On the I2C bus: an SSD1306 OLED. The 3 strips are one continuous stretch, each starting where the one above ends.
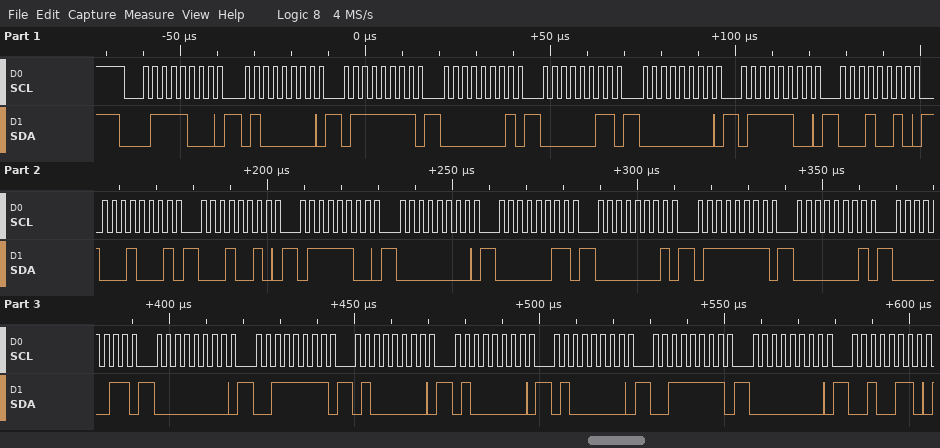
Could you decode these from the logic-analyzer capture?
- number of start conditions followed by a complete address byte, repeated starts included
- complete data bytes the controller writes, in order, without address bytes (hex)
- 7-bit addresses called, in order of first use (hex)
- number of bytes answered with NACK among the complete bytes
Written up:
1
40 7F 01 03 00 7C 12 11 12 7C 00 03 01 7F 01 03 00 3F 40 40 40 3F 00 26
0x3C
0
